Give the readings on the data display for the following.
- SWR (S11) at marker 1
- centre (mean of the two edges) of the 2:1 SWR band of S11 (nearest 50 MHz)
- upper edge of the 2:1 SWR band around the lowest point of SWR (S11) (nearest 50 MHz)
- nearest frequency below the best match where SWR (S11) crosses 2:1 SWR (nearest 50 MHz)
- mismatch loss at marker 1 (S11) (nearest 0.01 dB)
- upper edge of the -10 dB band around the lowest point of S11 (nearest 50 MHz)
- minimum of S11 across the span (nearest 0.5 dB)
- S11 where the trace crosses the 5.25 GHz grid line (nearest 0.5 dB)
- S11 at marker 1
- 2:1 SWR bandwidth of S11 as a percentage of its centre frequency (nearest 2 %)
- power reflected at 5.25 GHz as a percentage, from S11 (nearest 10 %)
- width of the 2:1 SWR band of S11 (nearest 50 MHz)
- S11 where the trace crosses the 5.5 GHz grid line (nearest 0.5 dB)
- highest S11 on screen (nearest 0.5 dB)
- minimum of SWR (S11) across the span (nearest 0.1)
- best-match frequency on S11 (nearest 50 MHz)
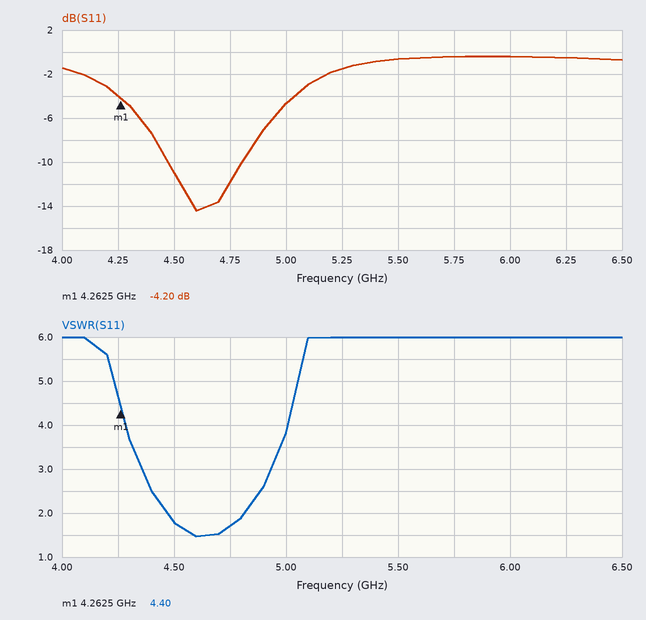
4.40
4.65 GHz
4.80 GHz
4.45 GHz
2.08 dB
4.80 GHz
-14.5 dB
-1.5 dB
-4.20 dB
8 %
70 %
350 MHz
-0.5 dB
-0.5 dB
1.5
4.60 GHz
